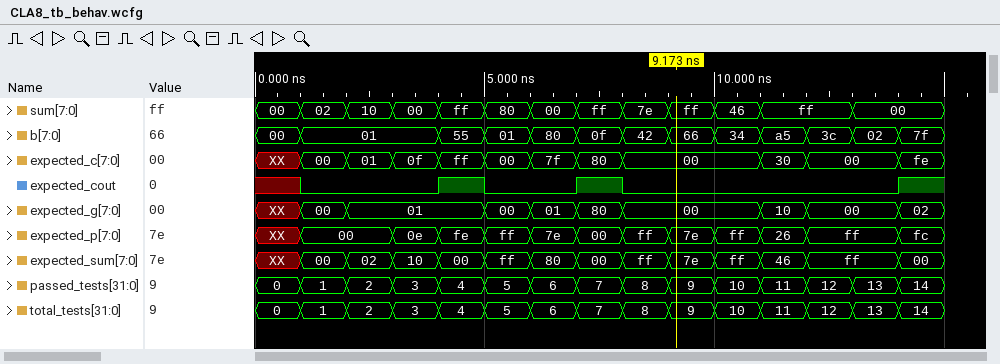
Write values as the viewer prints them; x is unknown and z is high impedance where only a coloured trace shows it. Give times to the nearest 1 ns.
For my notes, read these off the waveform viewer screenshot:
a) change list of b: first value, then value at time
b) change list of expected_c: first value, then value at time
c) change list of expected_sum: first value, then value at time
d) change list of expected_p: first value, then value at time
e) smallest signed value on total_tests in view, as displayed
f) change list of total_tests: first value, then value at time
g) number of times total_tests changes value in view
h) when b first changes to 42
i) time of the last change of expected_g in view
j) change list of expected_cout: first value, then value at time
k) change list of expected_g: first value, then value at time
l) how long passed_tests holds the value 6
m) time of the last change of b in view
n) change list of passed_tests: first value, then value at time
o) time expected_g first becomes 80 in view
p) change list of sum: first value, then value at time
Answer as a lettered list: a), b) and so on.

a) 00, 01 at 1 ns, 55 at 4 ns, 01 at 5 ns, 80 at 6 ns, 0f at 7 ns, 42 at 8 ns, 66 at 9 ns, 34 at 10 ns, a5 at 11 ns, 3c at 12 ns, 02 at 13 ns, 7f at 14 ns
b) XX, 00 at 1 ns, 01 at 2 ns, 0f at 3 ns, ff at 4 ns, 00 at 5 ns, 7f at 6 ns, 80 at 7 ns, 00 at 8 ns, 30 at 11 ns, 00 at 12 ns, fe at 14 ns
c) XX, 00 at 1 ns, 02 at 2 ns, 10 at 3 ns, 00 at 4 ns, ff at 5 ns, 80 at 6 ns, 00 at 7 ns, ff at 8 ns, 7e at 9 ns, ff at 10 ns, 46 at 11 ns, ff at 12 ns, 00 at 14 ns
d) XX, 00 at 1 ns, 0e at 3 ns, fe at 4 ns, ff at 5 ns, 7e at 6 ns, 00 at 7 ns, ff at 8 ns, 7e at 9 ns, ff at 10 ns, 26 at 11 ns, ff at 12 ns, fc at 14 ns
e) 0
f) 0, 1 at 1 ns, 2 at 2 ns, 3 at 3 ns, 4 at 4 ns, 5 at 5 ns, 6 at 6 ns, 7 at 7 ns, 8 at 8 ns, 9 at 9 ns, 10 at 10 ns, 11 at 11 ns, 12 at 12 ns, 13 at 13 ns, 14 at 14 ns
g) 14
h) 8 ns
i) 14 ns
j) x, 0 at 1 ns, 1 at 4 ns, 0 at 5 ns, 1 at 7 ns, 0 at 8 ns, 1 at 14 ns
k) XX, 00 at 1 ns, 01 at 2 ns, 00 at 5 ns, 01 at 6 ns, 80 at 7 ns, 00 at 8 ns, 10 at 11 ns, 00 at 12 ns, 02 at 14 ns
l) 1 ns
m) 14 ns
n) 0, 1 at 1 ns, 2 at 2 ns, 3 at 3 ns, 4 at 4 ns, 5 at 5 ns, 6 at 6 ns, 7 at 7 ns, 8 at 8 ns, 9 at 9 ns, 10 at 10 ns, 11 at 11 ns, 12 at 12 ns, 13 at 13 ns, 14 at 14 ns
o) 7 ns
p) 00, 02 at 1 ns, 10 at 2 ns, 00 at 3 ns, ff at 4 ns, 80 at 5 ns, 00 at 6 ns, ff at 7 ns, 7e at 8 ns, ff at 9 ns, 46 at 10 ns, ff at 11 ns, 00 at 13 ns
